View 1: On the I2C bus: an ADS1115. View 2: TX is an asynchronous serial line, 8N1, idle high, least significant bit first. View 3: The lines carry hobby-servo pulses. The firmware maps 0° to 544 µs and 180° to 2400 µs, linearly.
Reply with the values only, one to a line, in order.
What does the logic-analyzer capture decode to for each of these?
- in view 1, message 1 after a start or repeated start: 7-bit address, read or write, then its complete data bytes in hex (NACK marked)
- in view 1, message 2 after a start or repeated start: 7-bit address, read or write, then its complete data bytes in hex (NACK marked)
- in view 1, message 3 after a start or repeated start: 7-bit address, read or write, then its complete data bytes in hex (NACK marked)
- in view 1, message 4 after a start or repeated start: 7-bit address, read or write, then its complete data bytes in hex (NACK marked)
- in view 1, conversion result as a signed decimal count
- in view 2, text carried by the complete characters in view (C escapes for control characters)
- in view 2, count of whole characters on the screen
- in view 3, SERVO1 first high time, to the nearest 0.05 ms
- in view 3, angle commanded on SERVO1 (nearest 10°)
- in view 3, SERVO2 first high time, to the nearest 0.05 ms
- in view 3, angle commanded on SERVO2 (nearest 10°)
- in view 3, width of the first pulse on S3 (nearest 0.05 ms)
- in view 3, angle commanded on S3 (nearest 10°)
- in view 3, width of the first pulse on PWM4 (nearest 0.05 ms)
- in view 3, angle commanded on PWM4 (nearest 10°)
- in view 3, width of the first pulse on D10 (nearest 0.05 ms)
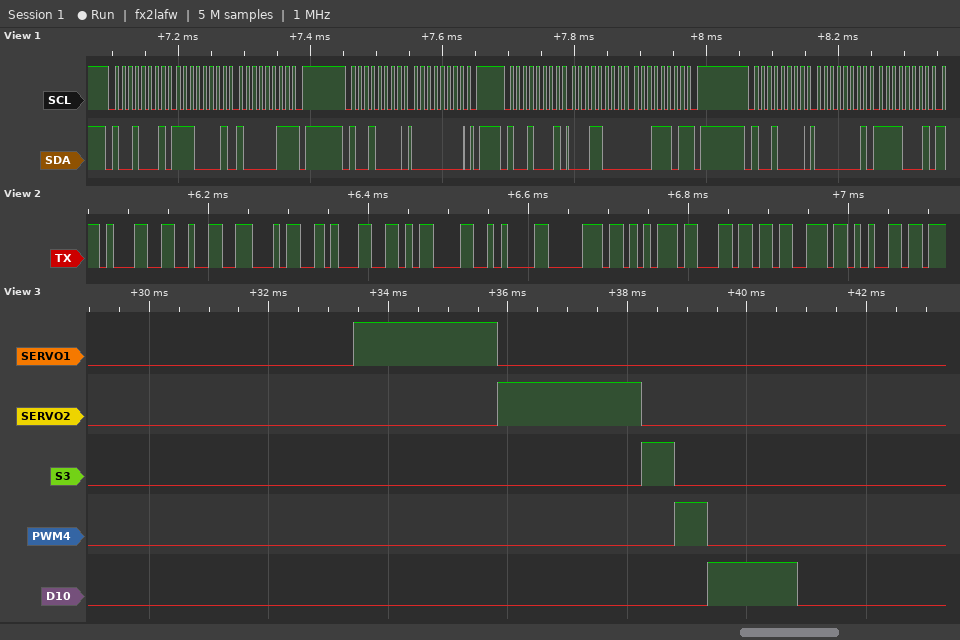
0x48 read: E1 83 NACK
0x48 write: 00
0x48 read: 18 1D NACK
0x48 write: 01 F1
6173
"1241\r\npulse"
11
2.40 ms
180°
2.40 ms
180°
0.55 ms
0°
0.55 ms
0°
1.50 ms
